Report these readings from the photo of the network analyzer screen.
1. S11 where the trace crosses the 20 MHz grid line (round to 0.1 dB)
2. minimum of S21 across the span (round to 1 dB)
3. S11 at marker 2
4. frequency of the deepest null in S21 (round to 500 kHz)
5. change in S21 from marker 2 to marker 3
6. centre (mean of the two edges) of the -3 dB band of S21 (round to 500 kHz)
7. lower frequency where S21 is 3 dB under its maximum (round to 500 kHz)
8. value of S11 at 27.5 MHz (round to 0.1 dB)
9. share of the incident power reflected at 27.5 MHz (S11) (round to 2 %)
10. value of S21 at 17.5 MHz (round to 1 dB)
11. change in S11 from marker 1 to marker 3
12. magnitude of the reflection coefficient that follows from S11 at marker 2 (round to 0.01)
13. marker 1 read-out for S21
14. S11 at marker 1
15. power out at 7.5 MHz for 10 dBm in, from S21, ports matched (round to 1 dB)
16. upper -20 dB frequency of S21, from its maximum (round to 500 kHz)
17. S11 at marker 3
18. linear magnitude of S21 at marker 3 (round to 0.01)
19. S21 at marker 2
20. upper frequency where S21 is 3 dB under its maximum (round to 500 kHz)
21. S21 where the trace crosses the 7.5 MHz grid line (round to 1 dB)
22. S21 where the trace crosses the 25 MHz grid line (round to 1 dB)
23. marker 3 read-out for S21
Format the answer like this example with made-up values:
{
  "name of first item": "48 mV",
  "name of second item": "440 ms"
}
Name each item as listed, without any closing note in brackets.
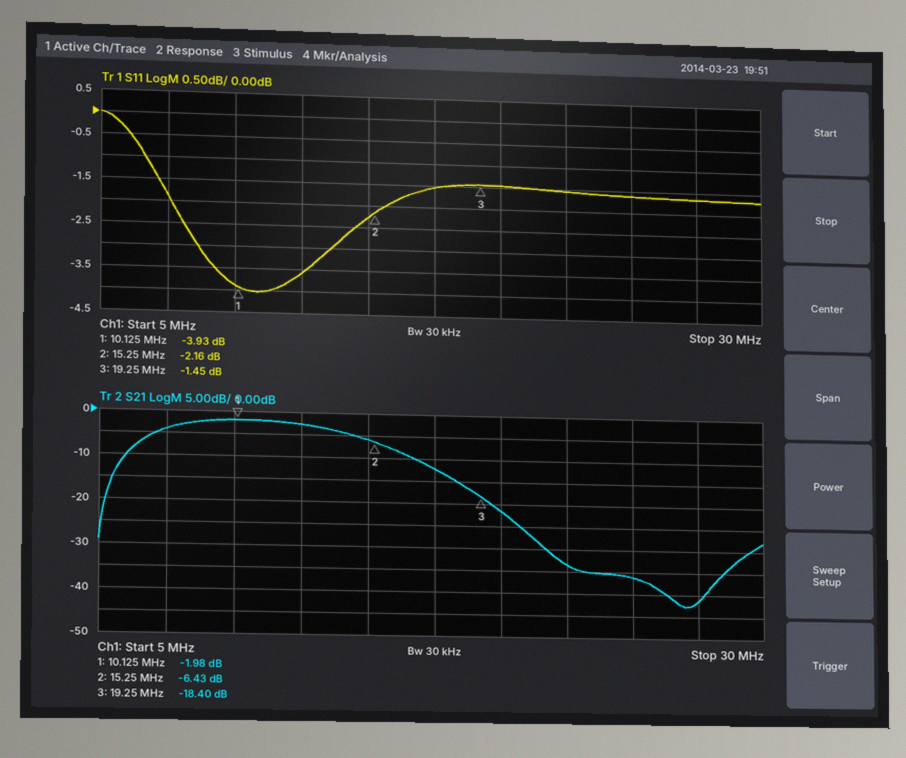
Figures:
{
  "S11 where the trace crosses the 20 MHz grid line": "-1.5 dB",
  "minimum of S21 across the span": "-43 dB",
  "S11 at marker 2": "-2.16 dB",
  "frequency of the deepest null in S21": "27.0 MHz",
  "change in S21 from marker 2 to marker 3": "-11.97 dB",
  "centre (mean of the two edges) of the -3 dB band of S21": "11.0 MHz",
  "lower frequency where S21 is 3 dB under its maximum": "7.0 MHz",
  "value of S11 at 27.5 MHz": "-1.7 dB",
  "share of the incident power reflected at 27.5 MHz (S11)": "68 %",
  "value of S21 at 17.5 MHz": "-12 dB",
  "change in S11 from marker 1 to marker 3": "2.48 dB",
  "magnitude of the reflection coefficient that follows from S11 at marker 2": "0.78",
  "marker 1 read-out for S21": "-1.98 dB",
  "S11 at marker 1": "-3.93 dB",
  "power out at 7.5 MHz for 10 dBm in, from S21, ports matched": "6 dBm",
  "upper -20 dB frequency of S21, from its maximum": "20.0 MHz",
  "S11 at marker 3": "-1.45 dB",
  "linear magnitude of S21 at marker 3": "0.12",
  "S21 at marker 2": "-6.43 dB",
  "upper frequency where S21 is 3 dB under its maximum": "14.5 MHz",
  "S21 where the trace crosses the 7.5 MHz grid line": "-4 dB",
  "S21 where the trace crosses the 25 MHz grid line": "-36 dB",
  "marker 3 read-out for S21": "-18.40 dB"
}
